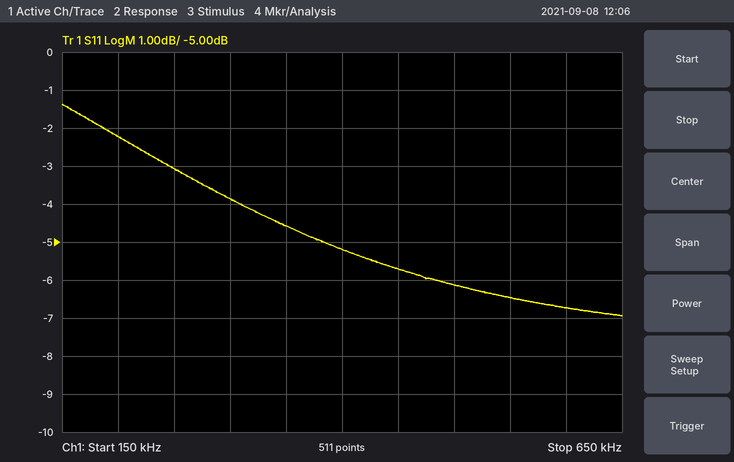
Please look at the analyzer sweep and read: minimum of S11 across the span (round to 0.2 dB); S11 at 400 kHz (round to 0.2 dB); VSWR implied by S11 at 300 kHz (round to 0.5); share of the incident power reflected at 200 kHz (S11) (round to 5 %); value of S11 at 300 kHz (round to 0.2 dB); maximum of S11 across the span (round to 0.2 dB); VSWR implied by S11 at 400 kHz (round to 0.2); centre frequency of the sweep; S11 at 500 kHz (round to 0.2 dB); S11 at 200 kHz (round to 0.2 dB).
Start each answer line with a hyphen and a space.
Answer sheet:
- -7.0 dB
- -5.2 dB
- 4.5
- 60 %
- -3.8 dB
- -1.4 dB
- 3.4
- 400 kHz
- -6.2 dB
- -2.2 dB
